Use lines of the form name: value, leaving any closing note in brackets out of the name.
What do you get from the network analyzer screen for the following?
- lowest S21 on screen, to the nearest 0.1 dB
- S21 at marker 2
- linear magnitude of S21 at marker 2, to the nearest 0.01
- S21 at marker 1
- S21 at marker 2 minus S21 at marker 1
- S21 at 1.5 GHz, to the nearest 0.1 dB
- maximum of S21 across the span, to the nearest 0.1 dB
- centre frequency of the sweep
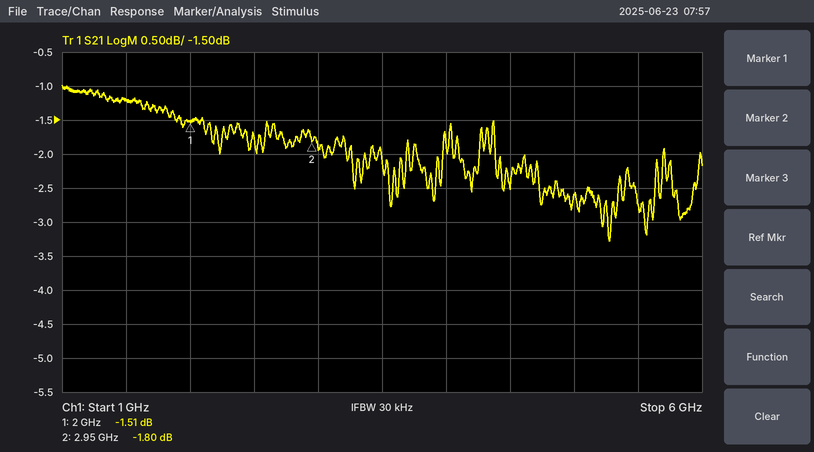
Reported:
lowest S21 on screen, to the nearest 0.1 dB: -3.3 dB
S21 at marker 2: -1.80 dB
linear magnitude of S21 at marker 2, to the nearest 0.01: 0.81
S21 at marker 1: -1.51 dB
S21 at marker 2 minus S21 at marker 1: -0.29 dB
S21 at 1.5 GHz, to the nearest 0.1 dB: -1.2 dB
maximum of S21 across the span, to the nearest 0.1 dB: -1.0 dB
centre frequency of the sweep: 3.5 GHz
